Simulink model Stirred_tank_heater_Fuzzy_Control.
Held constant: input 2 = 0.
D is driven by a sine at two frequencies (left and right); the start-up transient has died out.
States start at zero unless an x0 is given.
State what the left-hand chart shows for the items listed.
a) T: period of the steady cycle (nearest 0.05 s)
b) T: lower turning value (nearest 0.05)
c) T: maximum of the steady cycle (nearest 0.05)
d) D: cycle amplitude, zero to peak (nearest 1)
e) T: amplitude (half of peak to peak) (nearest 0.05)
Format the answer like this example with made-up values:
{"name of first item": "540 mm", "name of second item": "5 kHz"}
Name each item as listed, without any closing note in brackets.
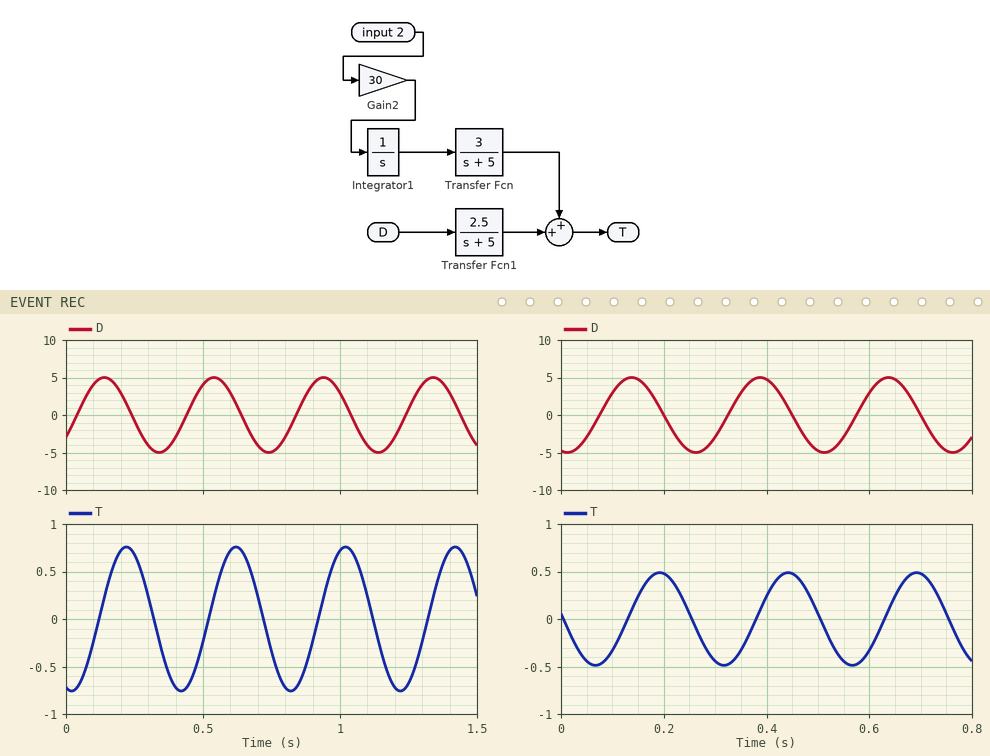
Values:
{"T: period of the steady cycle": "0.40 s", "T: lower turning value": "-0.75", "T: maximum of the steady cycle": "0.75", "D: cycle amplitude, zero to peak": "5", "T: amplitude (half of peak to peak)": "0.75"}
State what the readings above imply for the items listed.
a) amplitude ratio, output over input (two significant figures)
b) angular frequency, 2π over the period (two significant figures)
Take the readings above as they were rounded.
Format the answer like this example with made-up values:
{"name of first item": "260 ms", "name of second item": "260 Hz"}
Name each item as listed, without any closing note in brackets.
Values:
{"amplitude ratio, output over input": "0.15", "angular frequency, 2π over the period": "16 rad/s"}
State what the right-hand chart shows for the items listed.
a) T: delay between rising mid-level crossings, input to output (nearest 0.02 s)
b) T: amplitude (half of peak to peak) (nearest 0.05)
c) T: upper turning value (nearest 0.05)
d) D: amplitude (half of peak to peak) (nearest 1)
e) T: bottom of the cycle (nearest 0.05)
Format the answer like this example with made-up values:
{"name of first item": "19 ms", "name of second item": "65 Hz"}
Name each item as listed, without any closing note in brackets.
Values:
{"T: delay between rising mid-level crossings, input to output": "0.06 s", "T: amplitude (half of peak to peak)": "0.50", "T: upper turning value": "0.50", "D: amplitude (half of peak to peak)": "5", "T: bottom of the cycle": "-0.50"}
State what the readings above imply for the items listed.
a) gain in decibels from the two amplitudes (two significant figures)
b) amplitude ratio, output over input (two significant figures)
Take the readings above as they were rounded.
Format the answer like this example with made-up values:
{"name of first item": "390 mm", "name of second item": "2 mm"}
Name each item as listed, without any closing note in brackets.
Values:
{"gain in decibels from the two amplitudes": "-20 dB", "amplitude ratio, output over input": "0.10"}
